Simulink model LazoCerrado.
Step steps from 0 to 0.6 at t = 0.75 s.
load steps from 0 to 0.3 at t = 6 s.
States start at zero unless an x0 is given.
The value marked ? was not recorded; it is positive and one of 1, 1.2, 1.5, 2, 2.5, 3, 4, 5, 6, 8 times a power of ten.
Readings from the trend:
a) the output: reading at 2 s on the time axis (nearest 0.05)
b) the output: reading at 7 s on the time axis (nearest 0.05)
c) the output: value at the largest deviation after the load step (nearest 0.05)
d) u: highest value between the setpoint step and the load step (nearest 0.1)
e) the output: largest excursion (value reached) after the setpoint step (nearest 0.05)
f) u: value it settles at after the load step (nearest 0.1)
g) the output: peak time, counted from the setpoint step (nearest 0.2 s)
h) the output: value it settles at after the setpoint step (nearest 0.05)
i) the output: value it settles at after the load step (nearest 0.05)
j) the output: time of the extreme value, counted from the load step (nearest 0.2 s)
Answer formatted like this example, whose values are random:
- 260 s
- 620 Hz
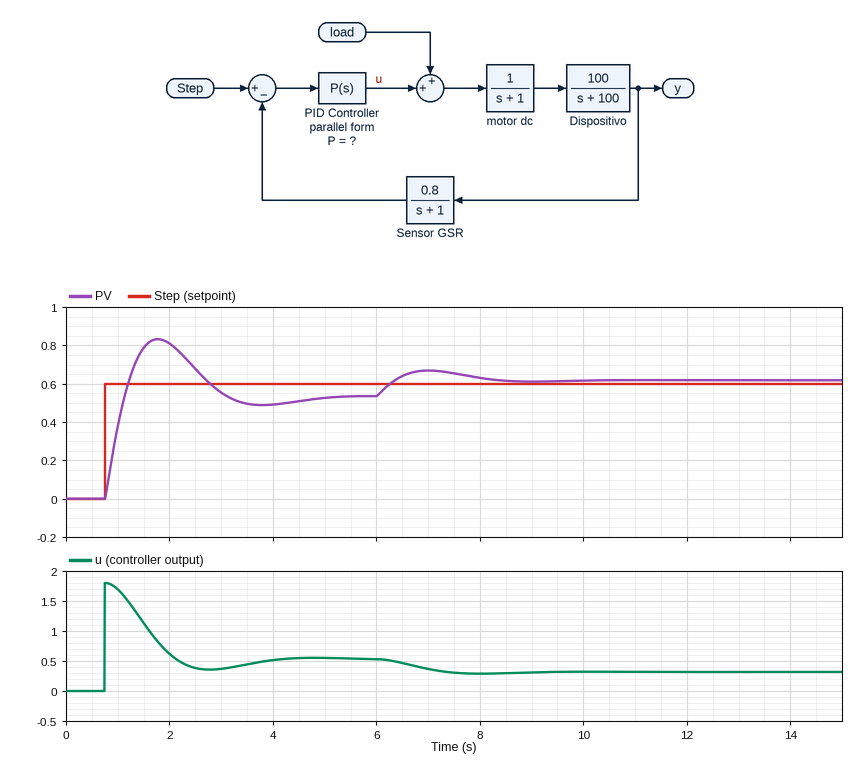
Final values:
- 0.80
- 0.65
- 0.65
- 1.8
- 0.85
- 0.3
- 1.0 s
- 0.55
- 0.60
- 1.0 s
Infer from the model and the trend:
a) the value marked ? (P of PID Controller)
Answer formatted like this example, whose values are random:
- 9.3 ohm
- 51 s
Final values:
- 3
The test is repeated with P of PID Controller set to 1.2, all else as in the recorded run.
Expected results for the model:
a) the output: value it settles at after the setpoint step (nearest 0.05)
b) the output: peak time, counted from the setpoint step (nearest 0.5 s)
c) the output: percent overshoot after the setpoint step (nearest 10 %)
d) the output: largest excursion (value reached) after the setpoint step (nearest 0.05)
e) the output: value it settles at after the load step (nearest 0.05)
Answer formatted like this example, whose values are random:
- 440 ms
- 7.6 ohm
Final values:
- 0.35
- 1.5 s
- 20 %
- 0.45
- 0.50
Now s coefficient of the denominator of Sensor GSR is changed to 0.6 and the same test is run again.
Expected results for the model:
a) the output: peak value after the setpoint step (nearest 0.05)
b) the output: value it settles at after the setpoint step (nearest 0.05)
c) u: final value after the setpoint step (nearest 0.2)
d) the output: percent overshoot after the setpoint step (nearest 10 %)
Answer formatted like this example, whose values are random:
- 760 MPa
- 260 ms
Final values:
- 0.75
- 0.55
- 0.6
- 40 %
